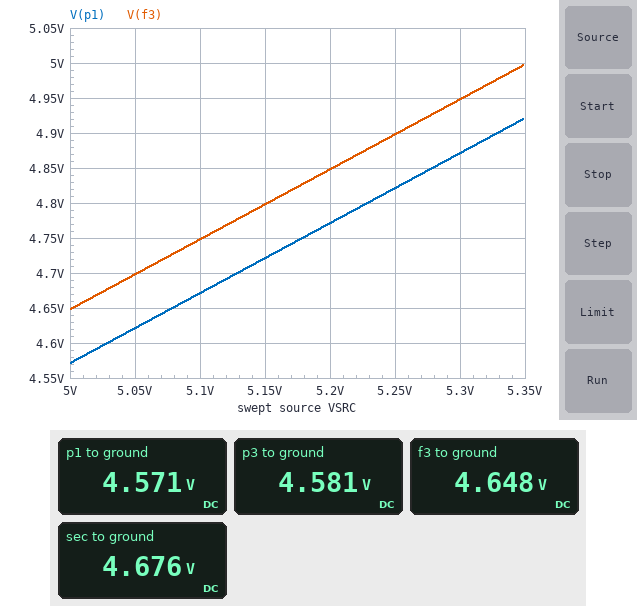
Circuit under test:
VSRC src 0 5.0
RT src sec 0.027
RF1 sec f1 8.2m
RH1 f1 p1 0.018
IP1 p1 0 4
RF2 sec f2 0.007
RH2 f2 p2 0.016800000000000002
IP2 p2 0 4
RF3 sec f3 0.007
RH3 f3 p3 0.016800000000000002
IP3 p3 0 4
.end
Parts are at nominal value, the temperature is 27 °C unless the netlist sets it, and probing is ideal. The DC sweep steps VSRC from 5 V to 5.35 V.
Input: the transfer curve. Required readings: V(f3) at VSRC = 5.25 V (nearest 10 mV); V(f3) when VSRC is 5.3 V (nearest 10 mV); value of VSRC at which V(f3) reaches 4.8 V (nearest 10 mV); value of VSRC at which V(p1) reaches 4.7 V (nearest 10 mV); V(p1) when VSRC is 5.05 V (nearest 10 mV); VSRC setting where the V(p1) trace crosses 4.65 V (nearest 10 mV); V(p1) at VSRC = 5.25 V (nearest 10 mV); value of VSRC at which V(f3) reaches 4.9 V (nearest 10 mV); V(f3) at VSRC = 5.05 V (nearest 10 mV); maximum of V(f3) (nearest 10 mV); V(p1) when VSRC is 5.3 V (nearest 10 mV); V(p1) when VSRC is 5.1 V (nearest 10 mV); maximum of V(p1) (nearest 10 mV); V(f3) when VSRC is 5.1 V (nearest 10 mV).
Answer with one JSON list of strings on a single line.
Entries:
["4.90 V", "4.95 V", "5.15 V", "5.13 V", "4.62 V", "5.08 V", "4.82 V", "5.25 V", "4.70 V", "5.00 V", "4.87 V", "4.67 V", "4.92 V", "4.75 V"]
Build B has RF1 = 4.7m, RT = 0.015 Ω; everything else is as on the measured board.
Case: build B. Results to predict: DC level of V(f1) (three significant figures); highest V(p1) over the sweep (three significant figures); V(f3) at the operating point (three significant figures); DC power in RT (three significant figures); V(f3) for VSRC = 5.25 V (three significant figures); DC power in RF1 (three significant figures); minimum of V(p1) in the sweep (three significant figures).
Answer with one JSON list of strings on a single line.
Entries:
["4.80 V", "5.08 V", "4.79 V", "2.16 W", "5.04 V", "75.2 mW", "4.73 V"]
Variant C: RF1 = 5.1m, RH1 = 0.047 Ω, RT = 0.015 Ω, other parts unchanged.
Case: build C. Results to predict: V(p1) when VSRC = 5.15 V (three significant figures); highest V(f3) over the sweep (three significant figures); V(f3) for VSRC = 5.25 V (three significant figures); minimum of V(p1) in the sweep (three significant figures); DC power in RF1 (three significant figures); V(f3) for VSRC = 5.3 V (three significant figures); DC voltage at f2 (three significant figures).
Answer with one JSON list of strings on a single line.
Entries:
["4.76 V", "5.14 V", "5.04 V", "4.61 V", "81.6 mW", "5.09 V", "4.79 V"]
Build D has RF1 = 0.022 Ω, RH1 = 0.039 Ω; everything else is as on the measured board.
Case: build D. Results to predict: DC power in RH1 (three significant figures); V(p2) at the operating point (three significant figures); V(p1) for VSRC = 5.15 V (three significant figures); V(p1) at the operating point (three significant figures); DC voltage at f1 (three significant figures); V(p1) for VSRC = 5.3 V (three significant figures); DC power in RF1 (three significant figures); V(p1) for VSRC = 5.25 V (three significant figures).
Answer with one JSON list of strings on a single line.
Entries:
["624 mW", "4.58 V", "4.58 V", "4.43 V", "4.59 V", "4.73 V", "352 mW", "4.68 V"]
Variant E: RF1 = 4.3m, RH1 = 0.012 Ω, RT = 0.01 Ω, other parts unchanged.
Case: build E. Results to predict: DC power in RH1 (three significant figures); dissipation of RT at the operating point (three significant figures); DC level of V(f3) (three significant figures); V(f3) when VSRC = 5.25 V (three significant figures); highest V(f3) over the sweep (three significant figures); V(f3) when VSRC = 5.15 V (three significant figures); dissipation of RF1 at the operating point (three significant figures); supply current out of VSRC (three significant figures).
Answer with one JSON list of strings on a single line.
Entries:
["192 mW", "1.44 W", "4.85 V", "5.10 V", "5.20 V", "5.00 V", "68.8 mW", "12.0 A"]
